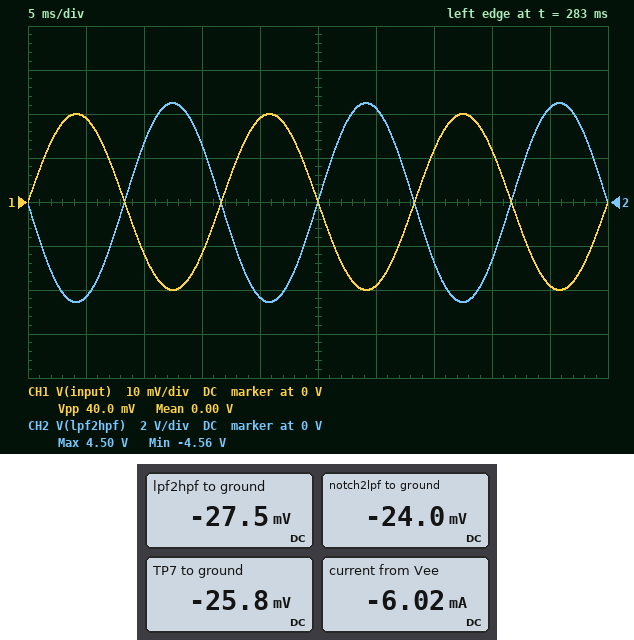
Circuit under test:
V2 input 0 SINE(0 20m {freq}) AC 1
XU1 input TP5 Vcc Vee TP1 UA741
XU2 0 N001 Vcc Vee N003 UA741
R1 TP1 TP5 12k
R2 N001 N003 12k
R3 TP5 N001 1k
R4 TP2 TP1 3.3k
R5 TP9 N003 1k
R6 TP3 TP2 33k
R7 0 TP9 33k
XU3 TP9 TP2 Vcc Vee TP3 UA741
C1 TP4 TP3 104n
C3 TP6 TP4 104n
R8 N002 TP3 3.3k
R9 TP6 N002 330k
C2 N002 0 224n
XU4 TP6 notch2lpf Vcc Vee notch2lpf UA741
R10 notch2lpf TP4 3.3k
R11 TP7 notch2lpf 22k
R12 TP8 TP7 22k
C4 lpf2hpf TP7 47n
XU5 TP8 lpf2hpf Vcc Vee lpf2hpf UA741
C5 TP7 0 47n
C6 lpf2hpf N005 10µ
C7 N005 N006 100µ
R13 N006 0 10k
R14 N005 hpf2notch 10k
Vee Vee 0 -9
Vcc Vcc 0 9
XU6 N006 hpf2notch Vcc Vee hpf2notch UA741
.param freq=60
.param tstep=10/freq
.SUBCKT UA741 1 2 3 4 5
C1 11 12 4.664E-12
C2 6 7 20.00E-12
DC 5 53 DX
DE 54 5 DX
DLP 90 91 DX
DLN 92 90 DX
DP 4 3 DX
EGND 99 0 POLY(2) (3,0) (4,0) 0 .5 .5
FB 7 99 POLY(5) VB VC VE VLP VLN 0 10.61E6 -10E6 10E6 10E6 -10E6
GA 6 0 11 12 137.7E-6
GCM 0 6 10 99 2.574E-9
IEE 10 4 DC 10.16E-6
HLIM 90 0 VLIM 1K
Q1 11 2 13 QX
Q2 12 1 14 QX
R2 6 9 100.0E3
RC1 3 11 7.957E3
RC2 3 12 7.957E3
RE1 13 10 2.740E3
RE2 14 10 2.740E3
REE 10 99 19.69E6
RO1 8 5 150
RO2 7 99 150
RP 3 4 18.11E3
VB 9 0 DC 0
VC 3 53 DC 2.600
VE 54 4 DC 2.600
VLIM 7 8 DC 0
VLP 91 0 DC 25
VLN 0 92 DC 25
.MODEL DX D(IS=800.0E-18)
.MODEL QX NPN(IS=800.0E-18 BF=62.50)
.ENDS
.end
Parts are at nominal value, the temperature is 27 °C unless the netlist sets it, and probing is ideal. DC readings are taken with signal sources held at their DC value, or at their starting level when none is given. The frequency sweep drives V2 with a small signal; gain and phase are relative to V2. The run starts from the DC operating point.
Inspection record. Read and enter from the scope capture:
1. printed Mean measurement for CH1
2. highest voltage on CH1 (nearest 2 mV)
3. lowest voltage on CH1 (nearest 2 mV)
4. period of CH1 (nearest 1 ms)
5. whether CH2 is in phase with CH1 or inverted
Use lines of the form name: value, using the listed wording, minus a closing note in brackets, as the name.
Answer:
printed Mean measurement for CH1: 0.00 V
highest voltage on CH1: 20 mV
lowest voltage on CH1: -20 mV
period of CH1: 17 ms
whether CH2 is in phase with CH1 or inverted: inverted
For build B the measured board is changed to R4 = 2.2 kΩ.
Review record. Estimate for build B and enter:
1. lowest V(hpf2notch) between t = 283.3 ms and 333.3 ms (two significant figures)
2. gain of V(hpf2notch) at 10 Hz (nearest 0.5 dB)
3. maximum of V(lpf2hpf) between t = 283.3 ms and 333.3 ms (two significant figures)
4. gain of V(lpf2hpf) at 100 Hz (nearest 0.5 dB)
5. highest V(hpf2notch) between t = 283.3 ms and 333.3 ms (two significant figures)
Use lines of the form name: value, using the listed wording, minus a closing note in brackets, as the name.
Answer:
lowest V(hpf2notch) between t = 283.3 ms and 333.3 ms: -6.4 V
gain of V(hpf2notch) at 10 Hz: 51.5 dB
maximum of V(lpf2hpf) between t = 283.3 ms and 333.3 ms: 6.3 V
gain of V(lpf2hpf) at 100 Hz: 50.0 dB
highest V(hpf2notch) between t = 283.3 ms and 333.3 ms: 6.4 V
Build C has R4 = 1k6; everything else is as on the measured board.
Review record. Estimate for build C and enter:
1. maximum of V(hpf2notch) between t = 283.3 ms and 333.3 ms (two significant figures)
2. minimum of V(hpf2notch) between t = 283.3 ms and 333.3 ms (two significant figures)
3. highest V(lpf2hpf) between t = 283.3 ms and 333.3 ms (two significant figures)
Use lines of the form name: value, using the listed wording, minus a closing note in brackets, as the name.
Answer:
maximum of V(hpf2notch) between t = 283.3 ms and 333.3 ms: 6.3 V
minimum of V(hpf2notch) between t = 283.3 ms and 333.3 ms: -6.2 V
highest V(lpf2hpf) between t = 283.3 ms and 333.3 ms: 6.2 V
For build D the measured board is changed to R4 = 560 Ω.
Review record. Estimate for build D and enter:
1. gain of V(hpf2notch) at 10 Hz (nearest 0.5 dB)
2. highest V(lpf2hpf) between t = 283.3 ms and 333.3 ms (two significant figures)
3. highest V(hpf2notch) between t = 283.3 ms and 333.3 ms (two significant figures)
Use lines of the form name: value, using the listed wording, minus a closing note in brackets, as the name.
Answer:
gain of V(hpf2notch) at 10 Hz: 63.0 dB
highest V(lpf2hpf) between t = 283.3 ms and 333.3 ms: 5.4 V
highest V(hpf2notch) between t = 283.3 ms and 333.3 ms: 5.5 V
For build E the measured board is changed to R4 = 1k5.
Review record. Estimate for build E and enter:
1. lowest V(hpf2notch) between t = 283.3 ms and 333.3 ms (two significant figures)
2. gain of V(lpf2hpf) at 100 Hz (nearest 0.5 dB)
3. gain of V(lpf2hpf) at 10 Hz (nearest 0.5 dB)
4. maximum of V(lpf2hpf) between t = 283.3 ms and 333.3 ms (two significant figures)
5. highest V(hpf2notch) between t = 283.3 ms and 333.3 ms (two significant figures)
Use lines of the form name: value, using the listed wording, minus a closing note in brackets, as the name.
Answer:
lowest V(hpf2notch) between t = 283.3 ms and 333.3 ms: -6.2 V
gain of V(lpf2hpf) at 100 Hz: 53.5 dB
gain of V(lpf2hpf) at 10 Hz: 55.0 dB
maximum of V(lpf2hpf) between t = 283.3 ms and 333.3 ms: 6.1 V
highest V(hpf2notch) between t = 283.3 ms and 333.3 ms: 6.2 V
